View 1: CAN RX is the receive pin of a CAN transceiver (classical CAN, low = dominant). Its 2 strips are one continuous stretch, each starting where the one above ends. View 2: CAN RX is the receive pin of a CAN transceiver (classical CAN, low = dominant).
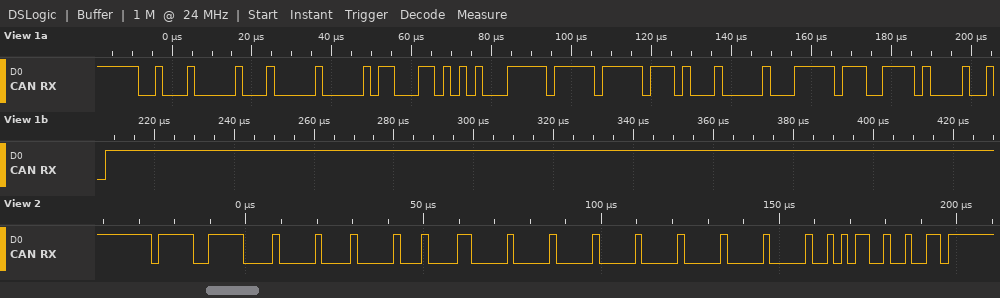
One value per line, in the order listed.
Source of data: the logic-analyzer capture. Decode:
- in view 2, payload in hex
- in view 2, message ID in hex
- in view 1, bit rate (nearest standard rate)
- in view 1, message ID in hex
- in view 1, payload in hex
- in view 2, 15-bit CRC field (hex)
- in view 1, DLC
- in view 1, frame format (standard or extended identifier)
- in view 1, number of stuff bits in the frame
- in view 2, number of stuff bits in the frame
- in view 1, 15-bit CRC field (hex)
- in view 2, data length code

02 01 0C 00 00 00 00 00
0x7DF
500 kbit/s
0x220
00 C6 A8 FF FF D1 00 FF
0x5649
8
standard
8
12
0x1E84
8
